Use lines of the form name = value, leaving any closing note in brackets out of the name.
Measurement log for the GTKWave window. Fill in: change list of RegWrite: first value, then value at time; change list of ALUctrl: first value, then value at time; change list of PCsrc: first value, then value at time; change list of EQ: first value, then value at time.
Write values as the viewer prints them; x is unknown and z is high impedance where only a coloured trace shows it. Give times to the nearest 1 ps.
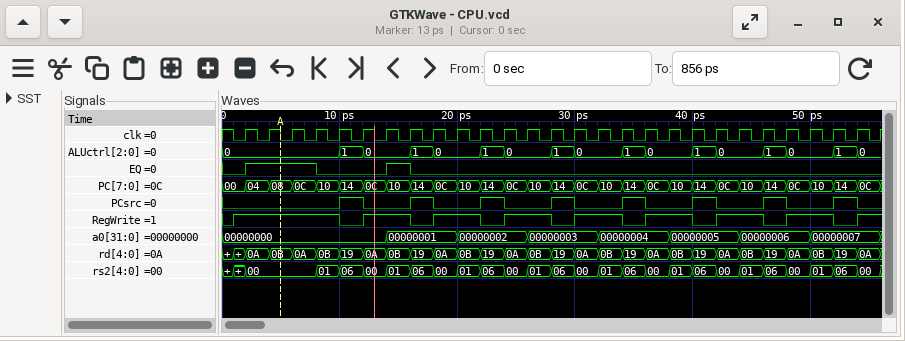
change list of RegWrite: first value, then value at time = 0, 1 at 1 ps, 0 at 10 ps, 1 at 12 ps, 0 at 16 ps, 1 at 18 ps, 0 at 22 ps, 1 at 24 ps, 0 at 28 ps, 1 at 30 ps, 0 at 34 ps, 1 at 36 ps, 0 at 40 ps, 1 at 42 ps, 0 at 46 ps, 1 at 48 ps, 0 at 52 ps, 1 at 54 ps
change list of ALUctrl: first value, then value at time = 0, 1 at 10 ps, 0 at 12 ps, 1 at 16 ps, 0 at 18 ps, 1 at 22 ps, 0 at 24 ps, 1 at 28 ps, 0 at 30 ps, 1 at 34 ps, 0 at 36 ps, 1 at 40 ps, 0 at 42 ps, 1 at 46 ps, 0 at 48 ps, 1 at 52 ps, 0 at 54 ps
change list of PCsrc: first value, then value at time = 0, 1 at 10 ps, 0 at 12 ps, 1 at 16 ps, 0 at 18 ps, 1 at 22 ps, 0 at 24 ps, 1 at 28 ps, 0 at 30 ps, 1 at 34 ps, 0 at 36 ps, 1 at 40 ps, 0 at 42 ps, 1 at 46 ps, 0 at 48 ps, 1 at 52 ps, 0 at 54 ps
change list of EQ: first value, then value at time = 0, 1 at 2 ps, 0 at 8 ps, 1 at 14 ps, 0 at 16 ps
